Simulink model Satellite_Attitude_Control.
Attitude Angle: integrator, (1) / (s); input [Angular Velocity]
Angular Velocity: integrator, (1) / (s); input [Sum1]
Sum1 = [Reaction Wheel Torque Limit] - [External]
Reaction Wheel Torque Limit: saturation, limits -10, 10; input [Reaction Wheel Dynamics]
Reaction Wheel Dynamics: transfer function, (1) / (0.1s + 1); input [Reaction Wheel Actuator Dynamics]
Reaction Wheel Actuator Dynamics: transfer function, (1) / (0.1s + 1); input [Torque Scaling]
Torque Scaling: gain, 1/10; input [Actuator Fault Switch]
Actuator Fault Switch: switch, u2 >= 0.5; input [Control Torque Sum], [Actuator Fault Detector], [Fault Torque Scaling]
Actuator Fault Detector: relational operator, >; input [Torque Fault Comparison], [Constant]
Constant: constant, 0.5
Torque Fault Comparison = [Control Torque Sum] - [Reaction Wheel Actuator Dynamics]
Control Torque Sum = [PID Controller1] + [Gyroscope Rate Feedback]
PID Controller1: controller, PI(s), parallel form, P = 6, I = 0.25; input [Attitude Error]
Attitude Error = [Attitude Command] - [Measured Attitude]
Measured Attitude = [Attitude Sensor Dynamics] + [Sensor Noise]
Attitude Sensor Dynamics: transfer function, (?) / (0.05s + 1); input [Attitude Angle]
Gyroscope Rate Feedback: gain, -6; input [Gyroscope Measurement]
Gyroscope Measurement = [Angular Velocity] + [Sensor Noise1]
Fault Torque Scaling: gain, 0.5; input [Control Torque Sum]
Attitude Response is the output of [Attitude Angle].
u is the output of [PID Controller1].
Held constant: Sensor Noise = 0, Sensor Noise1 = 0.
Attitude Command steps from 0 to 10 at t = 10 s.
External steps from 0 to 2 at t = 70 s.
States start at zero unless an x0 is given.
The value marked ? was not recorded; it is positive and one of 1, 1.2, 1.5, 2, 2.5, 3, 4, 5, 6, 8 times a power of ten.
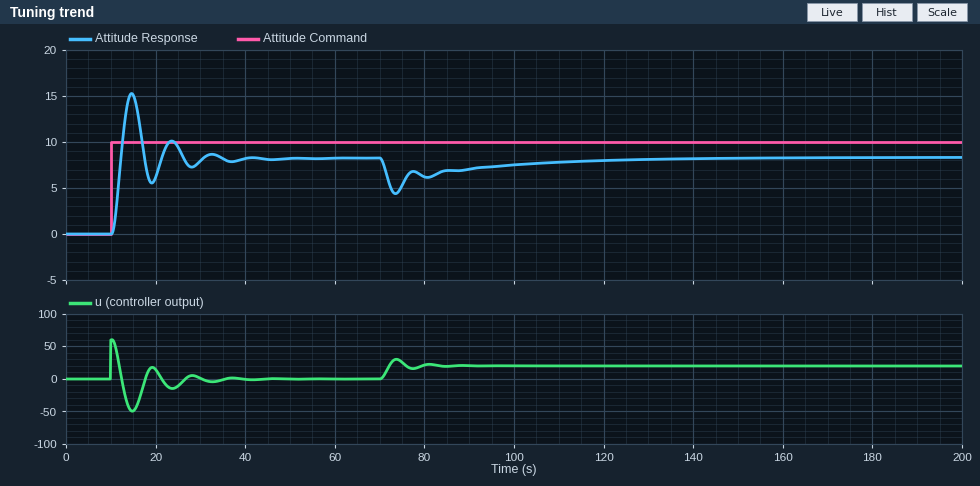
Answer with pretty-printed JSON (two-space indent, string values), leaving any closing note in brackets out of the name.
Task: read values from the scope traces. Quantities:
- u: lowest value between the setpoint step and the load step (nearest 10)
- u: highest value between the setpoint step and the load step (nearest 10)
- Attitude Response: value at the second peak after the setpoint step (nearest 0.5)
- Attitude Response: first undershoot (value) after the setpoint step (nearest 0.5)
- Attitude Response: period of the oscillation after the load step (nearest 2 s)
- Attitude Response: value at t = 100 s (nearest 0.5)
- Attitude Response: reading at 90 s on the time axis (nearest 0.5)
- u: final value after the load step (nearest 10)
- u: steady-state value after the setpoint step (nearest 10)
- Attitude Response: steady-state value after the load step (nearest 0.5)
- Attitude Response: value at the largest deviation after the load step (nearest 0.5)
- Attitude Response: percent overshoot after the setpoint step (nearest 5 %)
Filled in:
{
  "u: lowest value between the setpoint step and the load step": "-50",
  "u: highest value between the setpoint step and the load step": "60",
  "Attitude Response: value at the second peak after the setpoint step": "10.0",
  "Attitude Response: first undershoot (value) after the setpoint step": "5.5",
  "Attitude Response: period of the oscillation after the load step": "8 s",
  "Attitude Response: value at t = 100 s": "7.5",
  "Attitude Response: reading at 90 s on the time axis": "7.0",
  "u: final value after the load step": "20",
  "u: steady-state value after the setpoint step": "0",
  "Attitude Response: steady-state value after the load step": "8.5",
  "Attitude Response: value at the largest deviation after the load step": "4.5",
  "Attitude Response: percent overshoot after the setpoint step": "85 %"
}
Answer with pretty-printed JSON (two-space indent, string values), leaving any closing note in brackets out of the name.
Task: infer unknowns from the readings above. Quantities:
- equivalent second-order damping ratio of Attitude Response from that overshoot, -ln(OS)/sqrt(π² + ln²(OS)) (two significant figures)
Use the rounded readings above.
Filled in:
{
  "equivalent second-order damping ratio of Attitude Response from that overshoot, -ln(OS)/sqrt(π² + ln²(OS))": "0.052"
}
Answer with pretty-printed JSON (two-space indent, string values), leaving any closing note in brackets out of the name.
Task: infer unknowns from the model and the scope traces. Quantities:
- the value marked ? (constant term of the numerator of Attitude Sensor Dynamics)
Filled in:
{
  "the value marked ?": "1.2"
}
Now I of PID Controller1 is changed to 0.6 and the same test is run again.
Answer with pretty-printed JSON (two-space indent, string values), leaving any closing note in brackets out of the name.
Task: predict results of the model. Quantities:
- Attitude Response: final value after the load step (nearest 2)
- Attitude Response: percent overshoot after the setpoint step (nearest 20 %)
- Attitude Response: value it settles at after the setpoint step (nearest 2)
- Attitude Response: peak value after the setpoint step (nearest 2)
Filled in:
{
  "Attitude Response: final value after the load step": "8",
  "Attitude Response: percent overshoot after the setpoint step": "100 %",
  "Attitude Response: value it settles at after the setpoint step": "8",
  "Attitude Response: peak value after the setpoint step": "16"
}
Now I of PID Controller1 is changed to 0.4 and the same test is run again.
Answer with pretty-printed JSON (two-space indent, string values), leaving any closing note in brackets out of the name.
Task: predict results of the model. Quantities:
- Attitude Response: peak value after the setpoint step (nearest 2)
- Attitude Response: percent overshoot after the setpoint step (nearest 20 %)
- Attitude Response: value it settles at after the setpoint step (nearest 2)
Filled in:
{
  "Attitude Response: peak value after the setpoint step": "16",
  "Attitude Response: percent overshoot after the setpoint step": "80 %",
  "Attitude Response: value it settles at after the setpoint step": "8"
}
